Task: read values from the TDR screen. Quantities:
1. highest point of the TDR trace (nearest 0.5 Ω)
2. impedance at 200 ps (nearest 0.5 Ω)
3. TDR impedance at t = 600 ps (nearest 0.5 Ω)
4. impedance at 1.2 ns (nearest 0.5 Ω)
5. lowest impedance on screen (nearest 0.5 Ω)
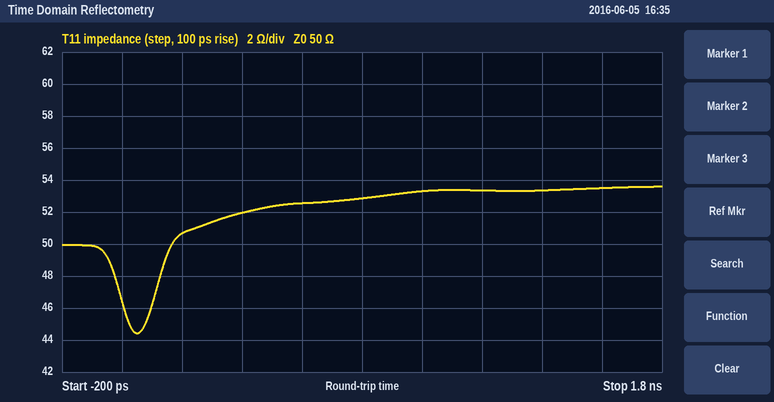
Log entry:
53.5 Ω
50.5 Ω
52.5 Ω
53.5 Ω
44.5 Ω
